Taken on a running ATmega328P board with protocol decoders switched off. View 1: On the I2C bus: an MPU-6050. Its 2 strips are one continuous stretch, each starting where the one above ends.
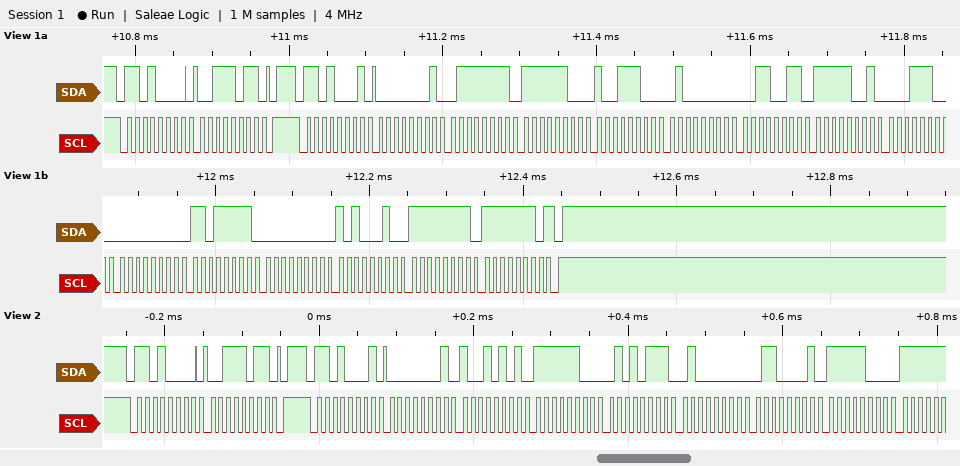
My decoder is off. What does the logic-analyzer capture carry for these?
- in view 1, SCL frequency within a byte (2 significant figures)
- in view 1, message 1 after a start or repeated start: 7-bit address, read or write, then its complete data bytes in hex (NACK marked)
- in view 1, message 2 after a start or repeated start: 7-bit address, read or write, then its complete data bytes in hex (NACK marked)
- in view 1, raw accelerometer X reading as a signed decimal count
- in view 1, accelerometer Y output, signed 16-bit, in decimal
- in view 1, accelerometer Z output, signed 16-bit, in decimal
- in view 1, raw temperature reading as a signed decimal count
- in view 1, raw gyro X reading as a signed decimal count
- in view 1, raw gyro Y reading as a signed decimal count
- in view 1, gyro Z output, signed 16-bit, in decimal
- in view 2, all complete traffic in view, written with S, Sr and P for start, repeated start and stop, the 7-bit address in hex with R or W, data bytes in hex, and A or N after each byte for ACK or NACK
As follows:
100 kHz
0x68 write: 3B
0x68 read: 01 7F FC 9C 40 33 F9 1C 00 DF 00 A2 FF FE NACK
383
-868
16435
-1764
223
162
-2
S 68W A 3B A P S 68R A 01 A 95 A FC A 57 A 40 A 61 A F8 A
